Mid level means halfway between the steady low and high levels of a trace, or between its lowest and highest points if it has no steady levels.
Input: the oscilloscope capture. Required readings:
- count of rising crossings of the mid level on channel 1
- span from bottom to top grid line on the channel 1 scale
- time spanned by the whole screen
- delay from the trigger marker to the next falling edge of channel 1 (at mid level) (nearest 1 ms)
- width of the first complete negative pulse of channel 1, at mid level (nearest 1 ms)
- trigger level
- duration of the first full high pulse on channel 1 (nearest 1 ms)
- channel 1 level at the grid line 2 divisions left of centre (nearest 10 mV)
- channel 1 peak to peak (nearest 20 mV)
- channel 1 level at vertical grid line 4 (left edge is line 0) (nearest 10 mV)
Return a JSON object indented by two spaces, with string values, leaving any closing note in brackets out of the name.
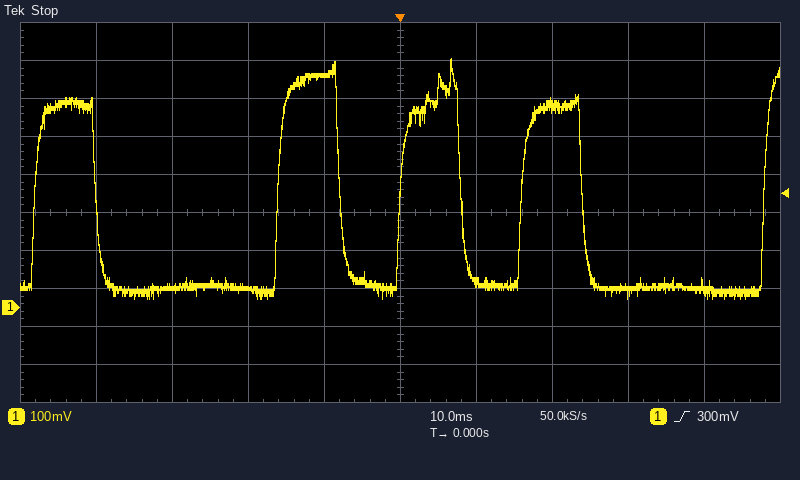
{
  "count of rising crossings of the mid level on channel 1": "5",
  "span from bottom to top grid line on the channel 1 scale": "1 V",
  "time spanned by the whole screen": "100 ms",
  "delay from the trigger marker to the next falling edge of channel 1 (at mid level)": "8 ms",
  "width of the first complete negative pulse of channel 1, at mid level": "24 ms",
  "trigger level": "300 mV",
  "duration of the first full high pulse on channel 1": "8 ms",
  "channel 1 level at the grid line 2 divisions left of centre": "50 mV",
  "channel 1 peak to peak": "640 mV",
  "channel 1 level at vertical grid line 4 (left edge is line 0)": "610 mV"
}
